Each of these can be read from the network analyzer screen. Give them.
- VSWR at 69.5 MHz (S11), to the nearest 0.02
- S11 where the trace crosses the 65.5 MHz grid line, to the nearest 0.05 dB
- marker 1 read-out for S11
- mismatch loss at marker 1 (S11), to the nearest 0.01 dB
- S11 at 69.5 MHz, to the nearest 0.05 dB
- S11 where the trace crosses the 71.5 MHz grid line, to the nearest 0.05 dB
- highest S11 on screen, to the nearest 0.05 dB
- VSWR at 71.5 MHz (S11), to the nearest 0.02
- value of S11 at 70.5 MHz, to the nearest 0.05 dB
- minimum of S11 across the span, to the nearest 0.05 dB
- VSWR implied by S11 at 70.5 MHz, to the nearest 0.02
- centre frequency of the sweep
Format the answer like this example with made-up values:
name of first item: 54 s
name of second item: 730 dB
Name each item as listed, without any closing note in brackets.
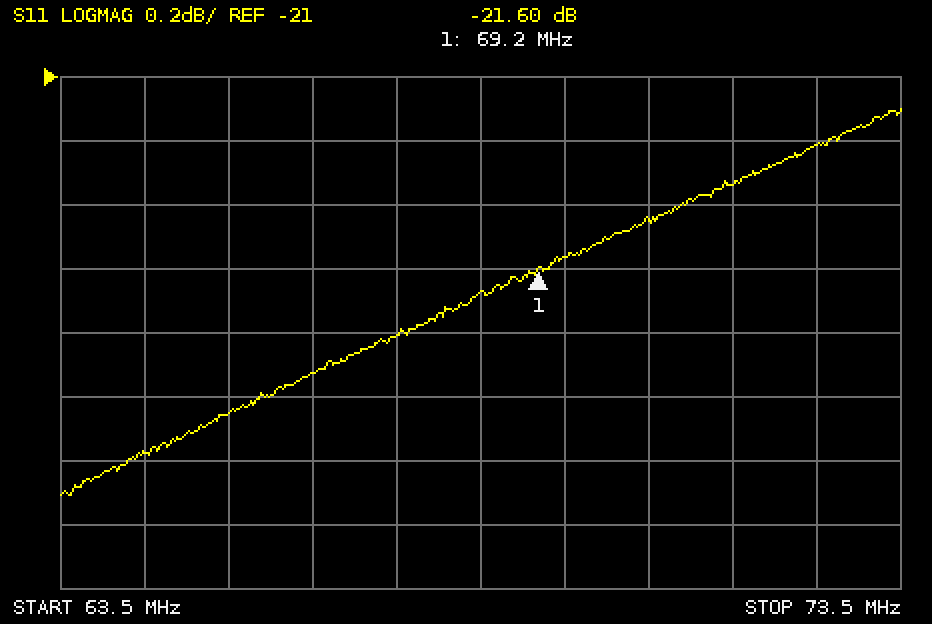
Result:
VSWR at 69.5 MHz (S11), to the nearest 0.02: 1.18
S11 where the trace crosses the 65.5 MHz grid line, to the nearest 0.05 dB: -22.05 dB
marker 1 read-out for S11: -21.60 dB
mismatch loss at marker 1 (S11), to the nearest 0.01 dB: 0.03 dB
S11 at 69.5 MHz, to the nearest 0.05 dB: -21.55 dB
S11 where the trace crosses the 71.5 MHz grid line, to the nearest 0.05 dB: -21.35 dB
highest S11 on screen, to the nearest 0.05 dB: -21.10 dB
VSWR at 71.5 MHz (S11), to the nearest 0.02: 1.18
value of S11 at 70.5 MHz, to the nearest 0.05 dB: -21.45 dB
minimum of S11 across the span, to the nearest 0.05 dB: -22.30 dB
VSWR implied by S11 at 70.5 MHz, to the nearest 0.02: 1.18
centre frequency of the sweep: 68.5 MHz
